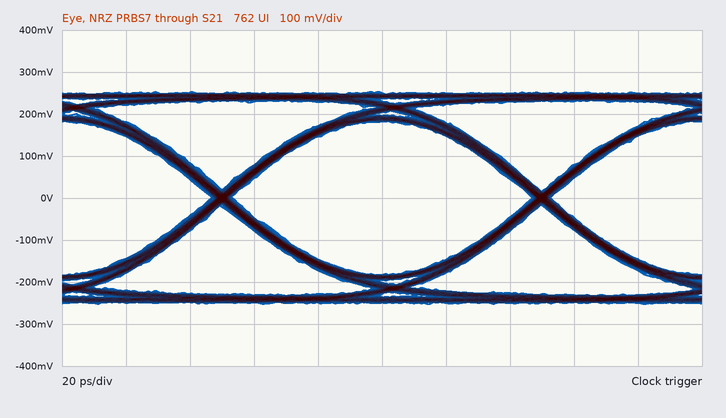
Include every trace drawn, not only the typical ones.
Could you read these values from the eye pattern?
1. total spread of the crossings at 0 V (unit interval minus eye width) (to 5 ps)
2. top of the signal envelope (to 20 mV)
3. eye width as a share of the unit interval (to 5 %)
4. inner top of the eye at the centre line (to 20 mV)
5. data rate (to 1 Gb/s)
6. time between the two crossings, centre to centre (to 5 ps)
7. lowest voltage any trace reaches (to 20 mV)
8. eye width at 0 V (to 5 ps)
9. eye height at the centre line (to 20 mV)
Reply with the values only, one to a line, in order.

5 ps
260 mV
95 %
180 mV
10 Gb/s
100 ps
-260 mV
95 ps
360 mV
